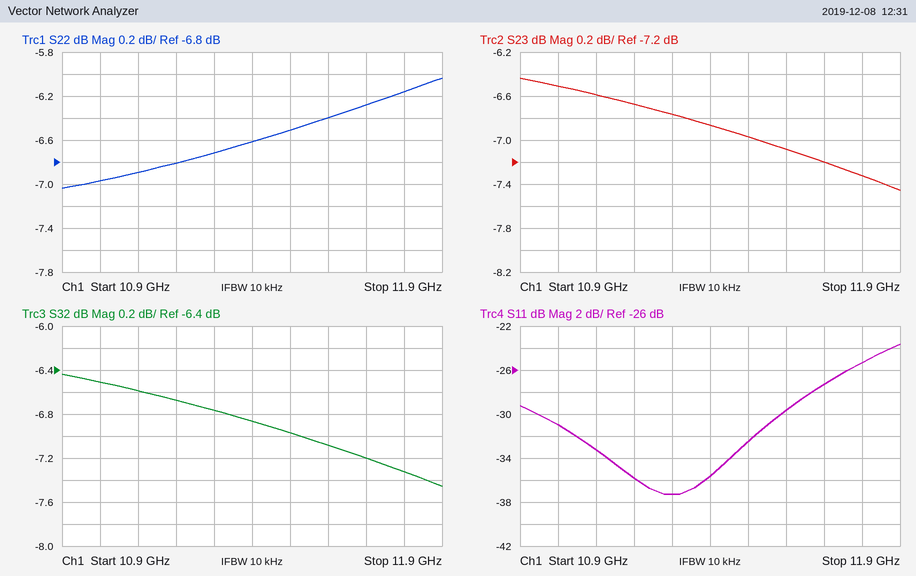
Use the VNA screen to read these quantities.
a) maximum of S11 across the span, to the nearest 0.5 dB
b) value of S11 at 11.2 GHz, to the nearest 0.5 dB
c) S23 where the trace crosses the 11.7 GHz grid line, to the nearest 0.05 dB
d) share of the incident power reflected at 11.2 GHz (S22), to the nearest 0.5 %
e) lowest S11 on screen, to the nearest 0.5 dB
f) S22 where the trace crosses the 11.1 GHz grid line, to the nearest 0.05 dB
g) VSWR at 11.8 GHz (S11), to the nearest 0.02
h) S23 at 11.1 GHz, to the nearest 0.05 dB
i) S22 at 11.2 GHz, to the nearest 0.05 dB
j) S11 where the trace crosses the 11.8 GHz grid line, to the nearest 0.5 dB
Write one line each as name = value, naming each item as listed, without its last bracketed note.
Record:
maximum of S11 across the span, to the nearest 0.5 dB = -23.5 dB
value of S11 at 11.2 GHz, to the nearest 0.5 dB = -36.0 dB
S23 where the trace crosses the 11.7 GHz grid line, to the nearest 0.05 dB = -7.20 dB
share of the incident power reflected at 11.2 GHz (S22), to the nearest 0.5 % = 21.0 %
lowest S11 on screen, to the nearest 0.5 dB = -37.5 dB
S22 where the trace crosses the 11.1 GHz grid line, to the nearest 0.05 dB = -6.90 dB
VSWR at 11.8 GHz (S11), to the nearest 0.02 = 1.12
S23 at 11.1 GHz, to the nearest 0.05 dB = -6.60 dB
S22 at 11.2 GHz, to the nearest 0.05 dB = -6.80 dB
S11 where the trace crosses the 11.8 GHz grid line, to the nearest 0.5 dB = -25.5 dB
